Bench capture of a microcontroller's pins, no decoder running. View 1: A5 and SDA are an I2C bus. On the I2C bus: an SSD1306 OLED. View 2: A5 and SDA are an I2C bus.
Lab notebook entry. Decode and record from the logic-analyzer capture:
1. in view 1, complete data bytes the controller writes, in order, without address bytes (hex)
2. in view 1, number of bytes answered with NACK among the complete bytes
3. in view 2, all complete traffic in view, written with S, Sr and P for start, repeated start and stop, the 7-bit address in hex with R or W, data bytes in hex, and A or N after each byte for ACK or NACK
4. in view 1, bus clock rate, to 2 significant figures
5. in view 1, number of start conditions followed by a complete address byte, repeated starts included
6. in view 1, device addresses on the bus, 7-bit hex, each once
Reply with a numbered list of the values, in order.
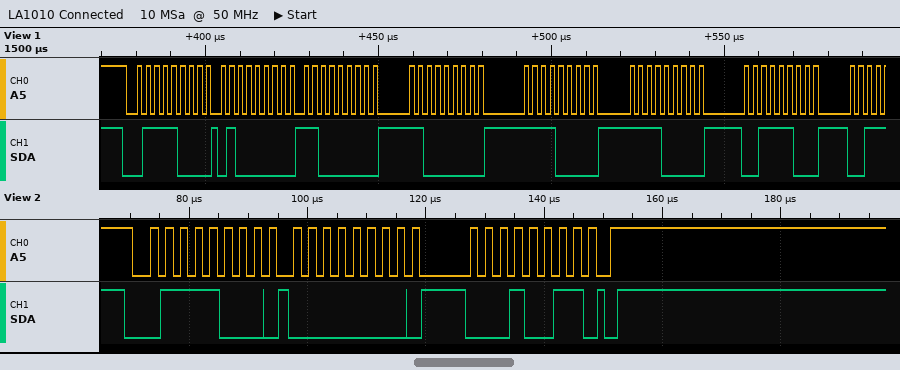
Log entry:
1. 40 C0 C0 F0 F0 3C
2. 0
3. S 3CW A 00 A 13 A P
4. 400 kHz
5. 1
6. 0x3C
